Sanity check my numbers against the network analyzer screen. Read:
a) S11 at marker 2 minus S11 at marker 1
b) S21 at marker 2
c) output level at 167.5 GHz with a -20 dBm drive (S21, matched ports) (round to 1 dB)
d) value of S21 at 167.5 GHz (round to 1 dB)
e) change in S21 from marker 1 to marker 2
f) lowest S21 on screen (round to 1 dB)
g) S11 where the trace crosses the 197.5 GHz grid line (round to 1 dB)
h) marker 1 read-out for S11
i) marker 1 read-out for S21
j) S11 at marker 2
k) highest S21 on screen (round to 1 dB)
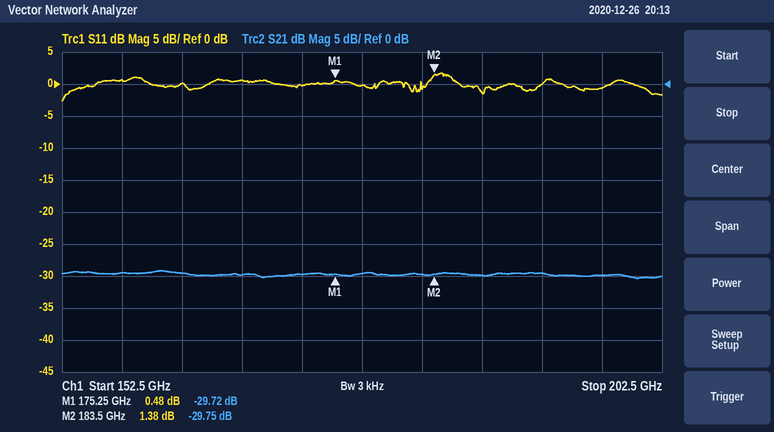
0.90 dB
-29.75 dB
-50 dBm
-30 dB
-0.03 dB
-30 dB
-1 dB
0.48 dB
-29.72 dB
1.38 dB
-29 dB
